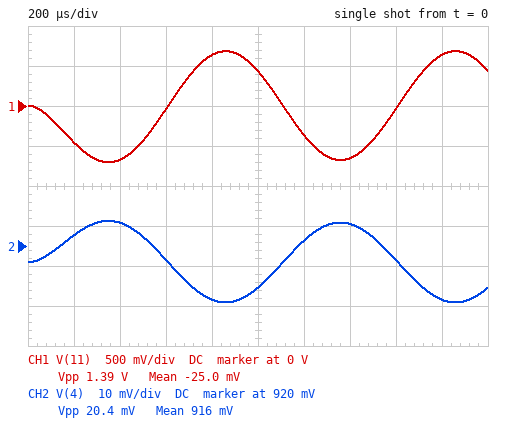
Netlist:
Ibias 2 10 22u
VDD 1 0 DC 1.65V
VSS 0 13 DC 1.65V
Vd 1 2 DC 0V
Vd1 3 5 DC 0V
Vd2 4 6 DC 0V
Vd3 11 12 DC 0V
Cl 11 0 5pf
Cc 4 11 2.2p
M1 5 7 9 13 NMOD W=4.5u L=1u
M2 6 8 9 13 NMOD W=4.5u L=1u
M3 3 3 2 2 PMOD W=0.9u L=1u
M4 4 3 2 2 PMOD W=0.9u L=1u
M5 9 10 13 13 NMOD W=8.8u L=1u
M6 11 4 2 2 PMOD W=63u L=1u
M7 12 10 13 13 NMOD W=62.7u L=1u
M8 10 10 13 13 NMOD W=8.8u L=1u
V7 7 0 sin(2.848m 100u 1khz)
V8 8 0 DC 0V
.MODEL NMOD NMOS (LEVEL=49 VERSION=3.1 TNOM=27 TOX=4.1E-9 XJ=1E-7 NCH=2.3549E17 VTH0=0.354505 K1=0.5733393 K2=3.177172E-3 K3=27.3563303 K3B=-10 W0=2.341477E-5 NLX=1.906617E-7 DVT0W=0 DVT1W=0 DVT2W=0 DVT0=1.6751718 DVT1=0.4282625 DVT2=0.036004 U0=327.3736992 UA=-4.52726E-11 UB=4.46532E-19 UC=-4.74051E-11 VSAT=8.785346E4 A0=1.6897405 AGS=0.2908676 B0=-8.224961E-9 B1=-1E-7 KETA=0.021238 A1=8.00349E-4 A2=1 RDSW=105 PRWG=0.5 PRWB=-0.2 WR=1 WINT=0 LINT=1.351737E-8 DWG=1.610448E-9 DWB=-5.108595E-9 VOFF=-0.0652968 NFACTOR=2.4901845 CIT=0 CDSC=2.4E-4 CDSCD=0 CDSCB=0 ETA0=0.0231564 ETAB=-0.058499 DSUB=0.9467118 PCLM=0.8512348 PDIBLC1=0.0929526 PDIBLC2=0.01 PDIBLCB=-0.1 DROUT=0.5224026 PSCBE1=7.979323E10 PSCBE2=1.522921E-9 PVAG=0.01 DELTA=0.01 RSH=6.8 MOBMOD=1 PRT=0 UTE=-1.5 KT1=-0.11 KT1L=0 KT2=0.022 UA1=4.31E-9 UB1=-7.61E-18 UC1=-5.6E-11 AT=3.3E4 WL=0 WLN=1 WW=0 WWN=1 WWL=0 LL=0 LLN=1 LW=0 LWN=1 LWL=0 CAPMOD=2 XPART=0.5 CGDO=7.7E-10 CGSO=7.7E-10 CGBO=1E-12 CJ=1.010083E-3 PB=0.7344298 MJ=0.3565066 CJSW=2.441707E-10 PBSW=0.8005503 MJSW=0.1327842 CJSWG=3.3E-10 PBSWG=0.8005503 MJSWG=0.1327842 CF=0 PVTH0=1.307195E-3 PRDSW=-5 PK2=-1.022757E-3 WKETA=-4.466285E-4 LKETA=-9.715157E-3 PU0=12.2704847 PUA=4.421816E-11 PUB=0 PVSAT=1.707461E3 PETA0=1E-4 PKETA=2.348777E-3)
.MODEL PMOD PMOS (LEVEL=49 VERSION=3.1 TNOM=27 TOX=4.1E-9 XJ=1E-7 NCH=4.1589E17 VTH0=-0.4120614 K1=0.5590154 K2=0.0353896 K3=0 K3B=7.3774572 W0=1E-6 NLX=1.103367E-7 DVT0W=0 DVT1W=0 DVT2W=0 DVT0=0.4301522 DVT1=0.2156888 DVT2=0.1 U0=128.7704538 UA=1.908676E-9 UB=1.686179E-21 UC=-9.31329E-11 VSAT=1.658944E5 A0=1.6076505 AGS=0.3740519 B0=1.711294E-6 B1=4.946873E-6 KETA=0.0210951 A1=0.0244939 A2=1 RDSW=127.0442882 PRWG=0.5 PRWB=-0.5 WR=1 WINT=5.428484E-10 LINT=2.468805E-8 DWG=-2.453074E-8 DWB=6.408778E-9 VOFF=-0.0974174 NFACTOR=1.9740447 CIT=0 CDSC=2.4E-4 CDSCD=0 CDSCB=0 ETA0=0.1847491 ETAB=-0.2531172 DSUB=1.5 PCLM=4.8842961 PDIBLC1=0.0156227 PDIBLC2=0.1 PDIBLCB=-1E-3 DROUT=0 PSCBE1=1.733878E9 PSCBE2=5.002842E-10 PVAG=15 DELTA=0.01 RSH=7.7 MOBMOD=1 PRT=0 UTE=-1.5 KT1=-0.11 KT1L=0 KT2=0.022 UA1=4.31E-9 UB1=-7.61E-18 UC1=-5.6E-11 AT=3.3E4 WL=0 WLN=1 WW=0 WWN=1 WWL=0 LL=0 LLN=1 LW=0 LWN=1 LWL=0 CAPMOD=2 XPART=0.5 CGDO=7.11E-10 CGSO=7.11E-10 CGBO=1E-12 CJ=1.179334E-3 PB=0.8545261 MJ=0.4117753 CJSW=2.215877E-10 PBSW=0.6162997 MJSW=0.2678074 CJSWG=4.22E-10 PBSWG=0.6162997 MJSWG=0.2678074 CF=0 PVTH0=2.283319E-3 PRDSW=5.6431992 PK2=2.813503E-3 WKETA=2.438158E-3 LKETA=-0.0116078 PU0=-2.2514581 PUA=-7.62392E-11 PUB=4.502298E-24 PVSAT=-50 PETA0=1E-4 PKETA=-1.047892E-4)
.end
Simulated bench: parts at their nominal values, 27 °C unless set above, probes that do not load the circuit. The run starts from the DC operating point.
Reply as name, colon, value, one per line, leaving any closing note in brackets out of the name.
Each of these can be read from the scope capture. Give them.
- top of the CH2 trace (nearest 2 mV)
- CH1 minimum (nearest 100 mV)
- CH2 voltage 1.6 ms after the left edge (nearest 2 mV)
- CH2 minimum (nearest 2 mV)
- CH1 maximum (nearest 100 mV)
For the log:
top of the CH2 trace: 926 mV
CH1 minimum: -700 mV
CH2 voltage 1.6 ms after the left edge: 916 mV
CH2 minimum: 906 mV
CH1 maximum: 700 mV
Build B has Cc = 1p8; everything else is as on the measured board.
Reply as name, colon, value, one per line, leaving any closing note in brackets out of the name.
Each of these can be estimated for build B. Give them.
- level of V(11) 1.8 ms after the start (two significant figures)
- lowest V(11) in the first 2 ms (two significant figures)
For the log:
level of V(11) 1.8 ms after the start: 710 mV
lowest V(11) in the first 2 ms: -740 mV
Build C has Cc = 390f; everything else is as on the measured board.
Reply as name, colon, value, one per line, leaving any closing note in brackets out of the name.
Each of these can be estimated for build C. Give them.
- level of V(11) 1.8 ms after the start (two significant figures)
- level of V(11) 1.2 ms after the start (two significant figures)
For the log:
level of V(11) 1.8 ms after the start: 860 mV
level of V(11) 1.2 ms after the start: -760 mV
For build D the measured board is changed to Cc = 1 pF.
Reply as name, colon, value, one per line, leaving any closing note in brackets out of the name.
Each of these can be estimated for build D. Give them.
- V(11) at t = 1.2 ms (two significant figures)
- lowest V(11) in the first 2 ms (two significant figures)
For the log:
V(11) at t = 1.2 ms: -630 mV
lowest V(11) in the first 2 ms: -810 mV
